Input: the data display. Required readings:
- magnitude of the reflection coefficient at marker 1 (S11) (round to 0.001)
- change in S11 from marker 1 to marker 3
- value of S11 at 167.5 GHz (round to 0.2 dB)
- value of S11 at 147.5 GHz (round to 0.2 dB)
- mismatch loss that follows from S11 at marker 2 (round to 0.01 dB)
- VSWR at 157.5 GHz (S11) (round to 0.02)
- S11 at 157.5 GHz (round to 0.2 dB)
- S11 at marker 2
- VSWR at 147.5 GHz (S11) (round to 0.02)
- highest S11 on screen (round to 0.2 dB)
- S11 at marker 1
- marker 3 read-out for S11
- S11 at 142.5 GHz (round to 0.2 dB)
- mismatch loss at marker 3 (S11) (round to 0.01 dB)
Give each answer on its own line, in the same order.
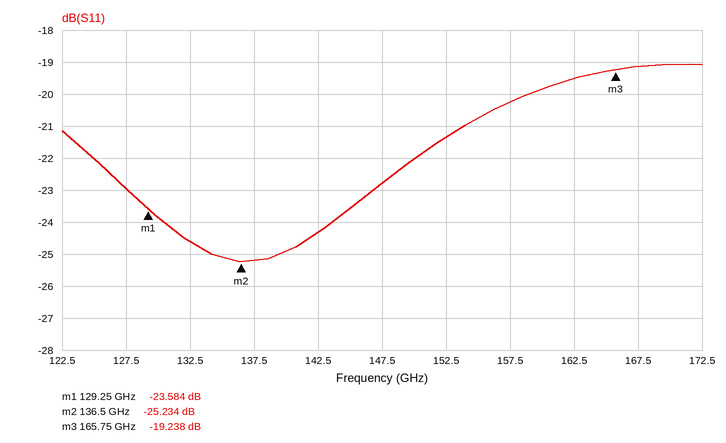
0.066
4.346 dB
-19.2 dB
-22.8 dB
0.01 dB
1.22
-20.2 dB
-25.234 dB
1.16
-19.0 dB
-23.584 dB
-19.238 dB
-24.4 dB
0.05 dB
